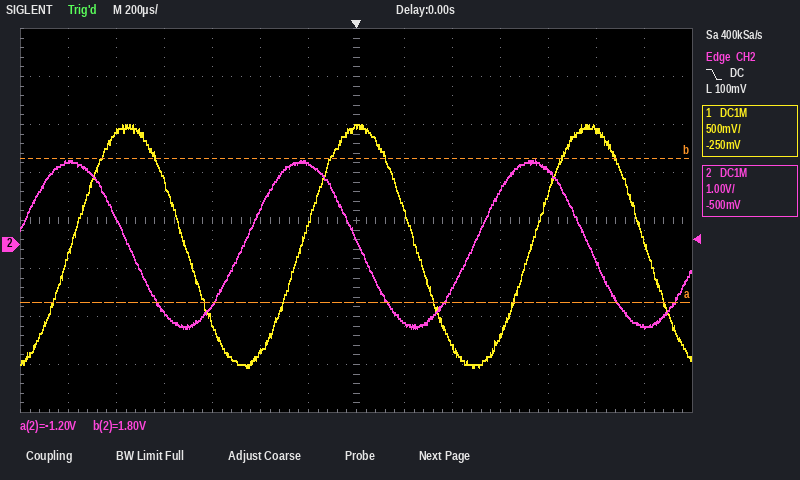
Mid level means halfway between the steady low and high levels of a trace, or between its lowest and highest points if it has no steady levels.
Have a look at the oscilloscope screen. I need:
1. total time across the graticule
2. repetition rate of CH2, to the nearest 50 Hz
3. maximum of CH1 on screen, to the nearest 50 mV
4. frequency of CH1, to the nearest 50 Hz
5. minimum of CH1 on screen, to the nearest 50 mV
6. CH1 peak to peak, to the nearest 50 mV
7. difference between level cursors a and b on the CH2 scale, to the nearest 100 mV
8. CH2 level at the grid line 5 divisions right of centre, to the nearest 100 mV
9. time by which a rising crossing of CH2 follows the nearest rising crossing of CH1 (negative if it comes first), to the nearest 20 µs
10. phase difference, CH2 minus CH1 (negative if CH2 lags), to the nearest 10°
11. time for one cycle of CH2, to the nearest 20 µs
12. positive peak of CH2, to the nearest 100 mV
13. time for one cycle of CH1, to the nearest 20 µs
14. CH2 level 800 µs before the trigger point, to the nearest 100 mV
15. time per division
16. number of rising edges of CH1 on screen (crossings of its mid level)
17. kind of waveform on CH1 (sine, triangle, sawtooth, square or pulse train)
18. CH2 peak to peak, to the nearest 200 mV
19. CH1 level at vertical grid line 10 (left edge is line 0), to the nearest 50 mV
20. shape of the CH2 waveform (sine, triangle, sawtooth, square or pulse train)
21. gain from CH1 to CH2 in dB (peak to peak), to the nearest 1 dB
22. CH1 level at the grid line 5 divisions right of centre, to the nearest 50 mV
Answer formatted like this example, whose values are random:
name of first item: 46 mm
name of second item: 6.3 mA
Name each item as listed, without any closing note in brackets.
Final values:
total time across the graticule: 2.8 ms
repetition rate of CH2, to the nearest 50 Hz: 1.05 kHz
maximum of CH1 on screen, to the nearest 50 mV: 1.25 V
frequency of CH1, to the nearest 50 Hz: 1.05 kHz
minimum of CH1 on screen, to the nearest 50 mV: -1.30 V
CH1 peak to peak, to the nearest 50 mV: 2.55 V
difference between level cursors a and b on the CH2 scale, to the nearest 100 mV: 3.0 V
CH2 level at the grid line 5 divisions right of centre, to the nearest 100 mV: -300 mV
time by which a rising crossing of CH2 follows the nearest rising crossing of CH1 (negative if it comes first), to the nearest 20 µs: -240 µs
phase difference, CH2 minus CH1 (negative if CH2 lags), to the nearest 10°: +90°
time for one cycle of CH2, to the nearest 20 µs: 960 µs
positive peak of CH2, to the nearest 100 mV: 1.8 V
time for one cycle of CH1, to the nearest 20 µs: 960 µs
CH2 level 800 µs before the trigger point, to the nearest 100 mV: -1.4 V
time per division: 200 µs
number of rising edges of CH1 on screen: 3
kind of waveform on CH1: sine
CH2 peak to peak, to the nearest 200 mV: 3.6 V
CH1 level at vertical grid line 10 (left edge is line 0), to the nearest 50 mV: -950 mV
shape of the CH2 waveform: sine
gain from CH1 to CH2 in dB (peak to peak), to the nearest 1 dB: 3 dB
CH1 level at the grid line 5 divisions right of centre, to the nearest 50 mV: 1.20 V
